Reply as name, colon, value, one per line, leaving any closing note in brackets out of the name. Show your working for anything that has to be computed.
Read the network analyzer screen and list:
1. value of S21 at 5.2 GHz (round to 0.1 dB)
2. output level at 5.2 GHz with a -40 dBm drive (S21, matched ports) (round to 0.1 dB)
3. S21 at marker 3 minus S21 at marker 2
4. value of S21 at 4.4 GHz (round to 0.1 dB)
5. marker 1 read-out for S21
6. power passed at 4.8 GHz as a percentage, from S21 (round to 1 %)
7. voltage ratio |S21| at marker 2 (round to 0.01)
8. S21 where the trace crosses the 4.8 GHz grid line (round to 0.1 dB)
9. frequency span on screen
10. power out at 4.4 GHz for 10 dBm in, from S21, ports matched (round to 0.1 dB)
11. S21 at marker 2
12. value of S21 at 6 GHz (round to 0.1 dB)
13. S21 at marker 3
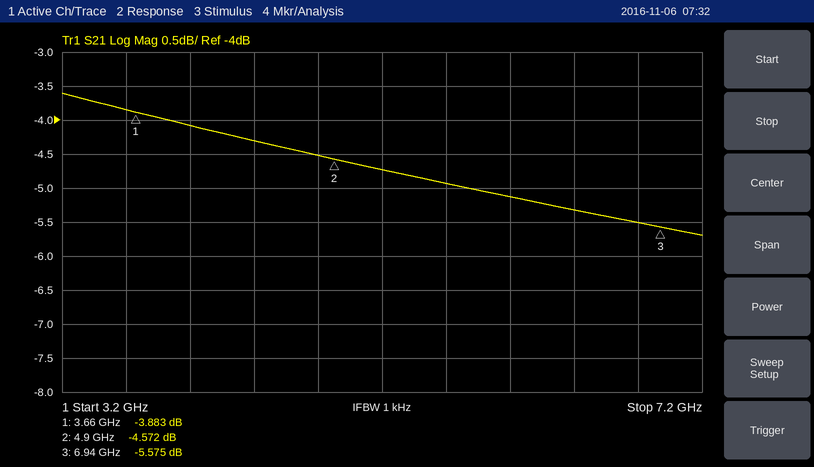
value of S21 at 5.2 GHz: -4.7 dB
output level at 5.2 GHz with a -40 dBm drive (S21, matched ports): -40 dBm + (-4.7 dB) = -44.7 dBm
S21 at marker 3 minus S21 at marker 2: -5.575 − (-4.572) = -1.003 dB
value of S21 at 4.4 GHz: -4.3 dB
marker 1 read-out for S21: -3.883 dB
power passed at 4.8 GHz as a percentage, from S21: 10^(-4.5/10) ≈ 35 %
voltage ratio |S21| at marker 2: 10^(-4.572/20) ≈ 0.59
S21 where the trace crosses the 4.8 GHz grid line: -4.5 dB
frequency span on screen: 4 GHz
power out at 4.4 GHz for 10 dBm in, from S21, ports matched: 10 dBm + (-4.3 dB) = 5.7 dBm
S21 at marker 2: -4.572 dB
value of S21 at 6 GHz: -5.1 dB
S21 at marker 3: -5.575 dB
